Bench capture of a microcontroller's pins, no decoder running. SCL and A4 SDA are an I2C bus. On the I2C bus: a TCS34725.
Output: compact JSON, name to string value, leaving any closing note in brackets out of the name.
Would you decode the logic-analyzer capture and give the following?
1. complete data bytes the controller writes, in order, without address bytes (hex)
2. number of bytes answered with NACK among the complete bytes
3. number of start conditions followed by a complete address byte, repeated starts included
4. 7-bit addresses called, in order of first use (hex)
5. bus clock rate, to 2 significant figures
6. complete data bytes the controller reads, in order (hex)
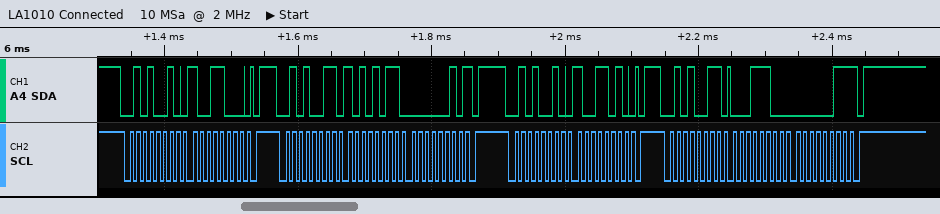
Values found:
{"complete data bytes the controller writes, in order, without address bytes": "98 9A", "number of bytes answered with NACK among the complete bytes": "2", "number of start conditions followed by a complete address byte, repeated starts included": "4", "7-bit addresses called, in order of first use": "0x29", "bus clock rate, to 2 significant figures": "100 kHz", "complete data bytes the controller reads, in order": "AB 02 1C 03"}
